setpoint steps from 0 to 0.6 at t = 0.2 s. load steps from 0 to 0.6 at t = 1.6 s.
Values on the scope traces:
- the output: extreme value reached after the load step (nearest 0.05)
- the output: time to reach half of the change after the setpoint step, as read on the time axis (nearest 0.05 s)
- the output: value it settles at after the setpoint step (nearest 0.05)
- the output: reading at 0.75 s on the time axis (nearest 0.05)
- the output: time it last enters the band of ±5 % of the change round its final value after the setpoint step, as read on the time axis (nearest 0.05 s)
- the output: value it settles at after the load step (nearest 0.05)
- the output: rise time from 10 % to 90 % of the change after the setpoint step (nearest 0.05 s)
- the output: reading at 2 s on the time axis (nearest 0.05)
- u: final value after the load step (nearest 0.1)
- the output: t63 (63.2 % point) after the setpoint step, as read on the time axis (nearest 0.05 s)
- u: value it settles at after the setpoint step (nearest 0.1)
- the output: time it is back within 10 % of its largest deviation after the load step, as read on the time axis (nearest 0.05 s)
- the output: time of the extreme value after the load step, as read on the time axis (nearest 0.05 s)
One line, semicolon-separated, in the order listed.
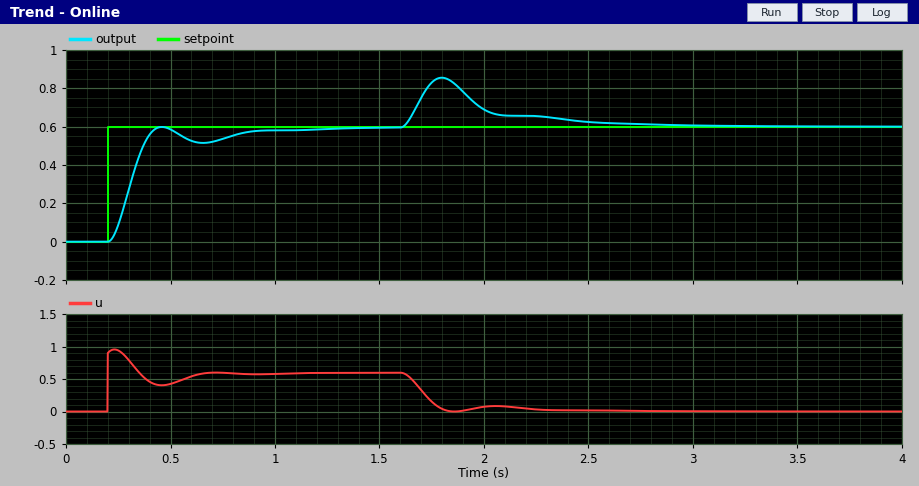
0.85; 0.30 s; 0.60; 0.55; 0.85 s; 0.60; 0.15 s; 0.70; 0.0; 0.35 s; 0.6; 2.50 s; 1.80 s
